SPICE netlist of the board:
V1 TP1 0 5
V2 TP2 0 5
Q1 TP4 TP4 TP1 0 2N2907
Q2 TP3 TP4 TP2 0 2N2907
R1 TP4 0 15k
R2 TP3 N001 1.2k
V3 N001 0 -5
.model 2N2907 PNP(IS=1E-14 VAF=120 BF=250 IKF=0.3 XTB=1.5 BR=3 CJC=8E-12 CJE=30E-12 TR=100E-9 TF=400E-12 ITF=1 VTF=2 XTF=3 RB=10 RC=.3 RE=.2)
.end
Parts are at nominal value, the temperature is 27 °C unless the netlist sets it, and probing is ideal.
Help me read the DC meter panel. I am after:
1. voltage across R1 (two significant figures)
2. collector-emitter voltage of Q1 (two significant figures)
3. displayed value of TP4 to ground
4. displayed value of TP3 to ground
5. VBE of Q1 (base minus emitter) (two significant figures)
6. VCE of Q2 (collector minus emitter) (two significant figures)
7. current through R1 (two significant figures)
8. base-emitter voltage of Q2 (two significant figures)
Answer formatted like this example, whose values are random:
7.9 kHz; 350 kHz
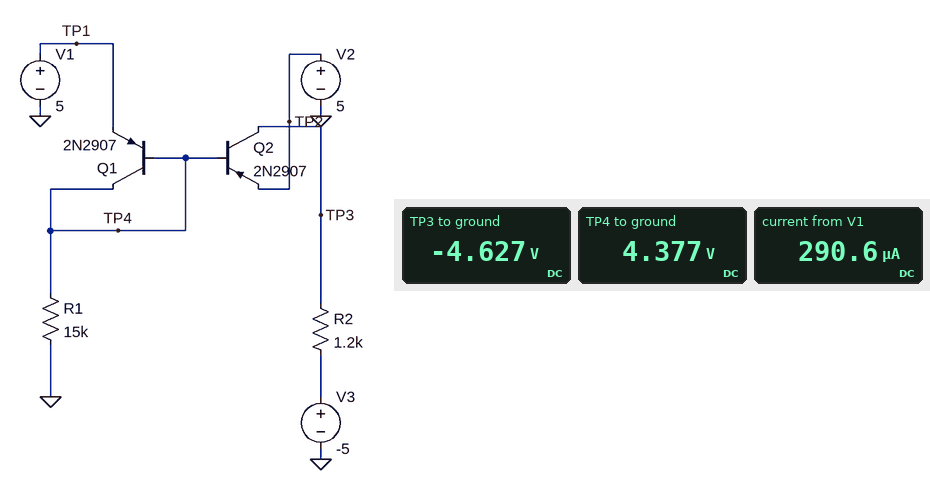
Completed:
4.4 V; -620 mV; 4.377 V; -4.627 V; -620 mV; -9.6 V; 290 µA; -620 mV
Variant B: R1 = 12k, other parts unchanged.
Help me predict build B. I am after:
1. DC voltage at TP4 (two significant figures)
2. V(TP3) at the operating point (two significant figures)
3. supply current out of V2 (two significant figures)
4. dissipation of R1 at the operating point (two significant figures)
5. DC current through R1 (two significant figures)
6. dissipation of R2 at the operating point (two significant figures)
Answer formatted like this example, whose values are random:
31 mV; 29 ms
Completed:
4.4 V; -4.5 V; 390 µA; 1.6 mW; 360 µA; 180 µW
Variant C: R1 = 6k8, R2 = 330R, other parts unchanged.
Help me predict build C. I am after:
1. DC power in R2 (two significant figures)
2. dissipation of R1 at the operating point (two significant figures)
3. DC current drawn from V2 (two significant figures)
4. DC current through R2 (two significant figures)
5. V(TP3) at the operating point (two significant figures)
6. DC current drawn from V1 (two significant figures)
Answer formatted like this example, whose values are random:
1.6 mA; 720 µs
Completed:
150 µW; 2.8 mW; 690 µA; 680 µA; -4.8 V; 640 µA
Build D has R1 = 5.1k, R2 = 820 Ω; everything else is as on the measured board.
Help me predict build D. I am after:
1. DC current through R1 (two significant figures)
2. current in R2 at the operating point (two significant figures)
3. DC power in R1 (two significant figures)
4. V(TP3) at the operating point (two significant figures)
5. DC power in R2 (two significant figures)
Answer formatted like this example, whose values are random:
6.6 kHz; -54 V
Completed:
850 µA; 910 µA; 3.7 mW; -4.3 V; 670 µW
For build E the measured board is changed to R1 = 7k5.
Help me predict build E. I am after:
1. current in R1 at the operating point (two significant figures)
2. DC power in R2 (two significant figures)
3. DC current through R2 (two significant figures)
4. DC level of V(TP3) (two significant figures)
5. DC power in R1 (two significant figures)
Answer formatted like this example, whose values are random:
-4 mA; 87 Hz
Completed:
580 µA; 460 µW; 620 µA; -4.3 V; 2.5 mW
